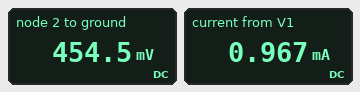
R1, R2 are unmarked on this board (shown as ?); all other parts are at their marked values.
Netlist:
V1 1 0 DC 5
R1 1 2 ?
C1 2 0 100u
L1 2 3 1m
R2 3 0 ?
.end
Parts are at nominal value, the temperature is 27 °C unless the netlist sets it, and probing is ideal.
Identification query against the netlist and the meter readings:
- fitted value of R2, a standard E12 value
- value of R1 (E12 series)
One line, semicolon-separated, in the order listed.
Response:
470 Ω; 4.7 kΩ
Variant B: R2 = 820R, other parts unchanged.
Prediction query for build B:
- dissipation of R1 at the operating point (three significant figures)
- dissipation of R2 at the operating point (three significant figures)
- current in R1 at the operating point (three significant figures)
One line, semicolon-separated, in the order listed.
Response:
3.86 mW; 673 µW; 906 µA
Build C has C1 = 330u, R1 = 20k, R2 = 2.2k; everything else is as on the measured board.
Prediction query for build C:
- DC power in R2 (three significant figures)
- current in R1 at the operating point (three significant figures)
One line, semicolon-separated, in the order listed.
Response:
112 µW; 225 µA
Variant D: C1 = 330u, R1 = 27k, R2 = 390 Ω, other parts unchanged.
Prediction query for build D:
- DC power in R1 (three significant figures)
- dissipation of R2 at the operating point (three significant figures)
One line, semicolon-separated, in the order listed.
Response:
900 µW; 13.0 µW
